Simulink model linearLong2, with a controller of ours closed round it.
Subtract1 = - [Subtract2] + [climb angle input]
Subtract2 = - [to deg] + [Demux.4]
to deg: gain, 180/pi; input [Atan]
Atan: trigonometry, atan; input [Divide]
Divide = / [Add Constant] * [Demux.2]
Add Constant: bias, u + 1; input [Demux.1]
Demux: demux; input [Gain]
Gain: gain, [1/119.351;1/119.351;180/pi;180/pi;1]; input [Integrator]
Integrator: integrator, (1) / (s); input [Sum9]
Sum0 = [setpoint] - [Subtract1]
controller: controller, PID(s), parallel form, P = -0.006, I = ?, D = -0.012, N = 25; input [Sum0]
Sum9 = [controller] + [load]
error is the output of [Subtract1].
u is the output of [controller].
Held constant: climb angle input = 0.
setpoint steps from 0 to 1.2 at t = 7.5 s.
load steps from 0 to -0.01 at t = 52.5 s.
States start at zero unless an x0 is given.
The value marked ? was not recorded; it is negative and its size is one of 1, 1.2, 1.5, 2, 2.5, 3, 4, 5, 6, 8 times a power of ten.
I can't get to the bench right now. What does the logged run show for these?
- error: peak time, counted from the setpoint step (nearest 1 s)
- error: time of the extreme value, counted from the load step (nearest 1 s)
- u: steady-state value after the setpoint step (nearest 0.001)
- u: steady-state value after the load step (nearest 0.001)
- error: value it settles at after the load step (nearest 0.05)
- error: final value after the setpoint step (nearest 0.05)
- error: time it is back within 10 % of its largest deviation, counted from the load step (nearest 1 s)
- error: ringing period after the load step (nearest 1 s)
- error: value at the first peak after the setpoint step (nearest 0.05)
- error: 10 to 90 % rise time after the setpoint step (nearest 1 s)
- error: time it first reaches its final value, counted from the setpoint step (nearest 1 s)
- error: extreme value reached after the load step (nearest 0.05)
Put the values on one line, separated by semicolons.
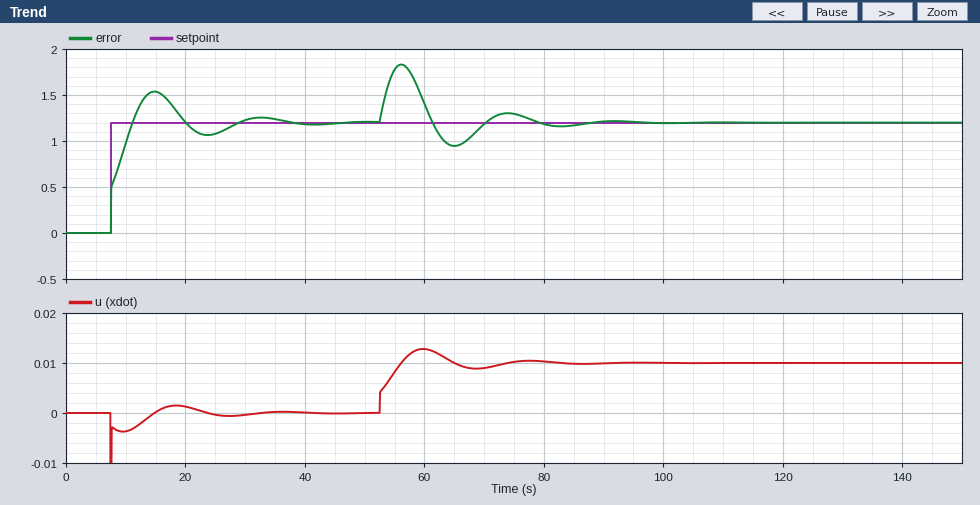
7 s; 4 s; 0.000; 0.010; 1.20; 1.20; 24 s; 18 s; 1.55; 3 s; 4 s; 1.85
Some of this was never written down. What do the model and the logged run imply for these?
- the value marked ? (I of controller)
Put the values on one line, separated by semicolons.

-0.004
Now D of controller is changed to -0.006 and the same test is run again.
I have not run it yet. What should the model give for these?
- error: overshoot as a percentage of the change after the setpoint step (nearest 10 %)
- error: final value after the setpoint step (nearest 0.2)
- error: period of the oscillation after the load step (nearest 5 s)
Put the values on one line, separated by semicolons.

30 %; 1.2; 15 s
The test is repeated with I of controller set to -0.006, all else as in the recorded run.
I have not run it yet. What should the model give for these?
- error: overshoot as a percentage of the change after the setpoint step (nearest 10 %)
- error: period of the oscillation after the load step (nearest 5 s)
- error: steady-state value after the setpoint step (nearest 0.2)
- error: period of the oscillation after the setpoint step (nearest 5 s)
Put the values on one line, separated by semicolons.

30 %; 15 s; 1.2; 15 s
